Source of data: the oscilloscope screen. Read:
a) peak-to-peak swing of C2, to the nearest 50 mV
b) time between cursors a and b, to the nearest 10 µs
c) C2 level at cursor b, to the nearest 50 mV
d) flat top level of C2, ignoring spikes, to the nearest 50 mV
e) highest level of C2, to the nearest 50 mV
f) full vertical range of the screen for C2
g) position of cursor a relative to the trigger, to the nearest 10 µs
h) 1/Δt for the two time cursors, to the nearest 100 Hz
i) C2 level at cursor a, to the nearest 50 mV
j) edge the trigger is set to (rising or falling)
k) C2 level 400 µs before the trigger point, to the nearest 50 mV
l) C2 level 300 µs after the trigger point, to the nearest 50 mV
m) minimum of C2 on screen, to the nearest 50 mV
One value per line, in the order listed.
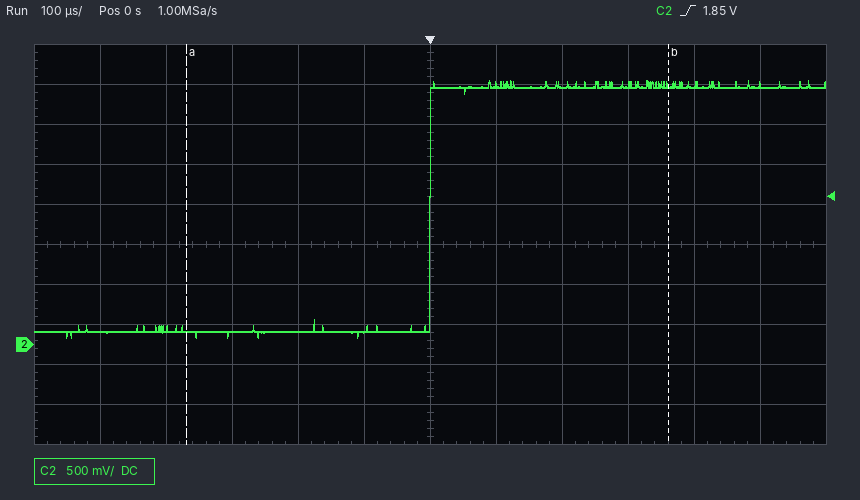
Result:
3.20 V
730 µs
3.25 V
3.20 V
3.30 V
5 V
-370 µs
1.4 kHz
150 mV
rising
200 mV
3.25 V
100 mV
